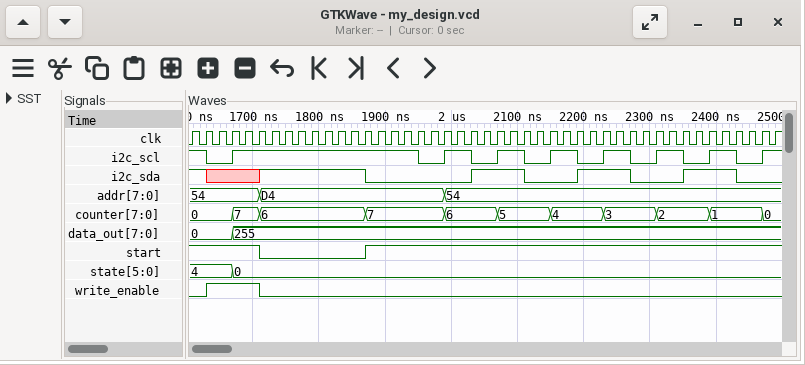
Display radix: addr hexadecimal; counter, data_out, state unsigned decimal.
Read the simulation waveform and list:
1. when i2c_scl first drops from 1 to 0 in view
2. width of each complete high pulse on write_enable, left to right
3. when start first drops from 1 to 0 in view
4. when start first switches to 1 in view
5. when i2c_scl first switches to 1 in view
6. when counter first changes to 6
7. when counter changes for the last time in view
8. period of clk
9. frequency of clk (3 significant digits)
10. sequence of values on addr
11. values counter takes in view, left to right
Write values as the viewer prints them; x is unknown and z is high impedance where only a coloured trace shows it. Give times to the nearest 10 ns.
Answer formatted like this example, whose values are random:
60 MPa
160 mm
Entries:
1630 ns
80 ns
1710 ns
1870 ns
1670 ns
1710 ns
2470 ns
20 ns
50.0 MHz
54, D4, 54
0, 7, 6, 7, 6, 5, 4, 3, 2, 1, 0
